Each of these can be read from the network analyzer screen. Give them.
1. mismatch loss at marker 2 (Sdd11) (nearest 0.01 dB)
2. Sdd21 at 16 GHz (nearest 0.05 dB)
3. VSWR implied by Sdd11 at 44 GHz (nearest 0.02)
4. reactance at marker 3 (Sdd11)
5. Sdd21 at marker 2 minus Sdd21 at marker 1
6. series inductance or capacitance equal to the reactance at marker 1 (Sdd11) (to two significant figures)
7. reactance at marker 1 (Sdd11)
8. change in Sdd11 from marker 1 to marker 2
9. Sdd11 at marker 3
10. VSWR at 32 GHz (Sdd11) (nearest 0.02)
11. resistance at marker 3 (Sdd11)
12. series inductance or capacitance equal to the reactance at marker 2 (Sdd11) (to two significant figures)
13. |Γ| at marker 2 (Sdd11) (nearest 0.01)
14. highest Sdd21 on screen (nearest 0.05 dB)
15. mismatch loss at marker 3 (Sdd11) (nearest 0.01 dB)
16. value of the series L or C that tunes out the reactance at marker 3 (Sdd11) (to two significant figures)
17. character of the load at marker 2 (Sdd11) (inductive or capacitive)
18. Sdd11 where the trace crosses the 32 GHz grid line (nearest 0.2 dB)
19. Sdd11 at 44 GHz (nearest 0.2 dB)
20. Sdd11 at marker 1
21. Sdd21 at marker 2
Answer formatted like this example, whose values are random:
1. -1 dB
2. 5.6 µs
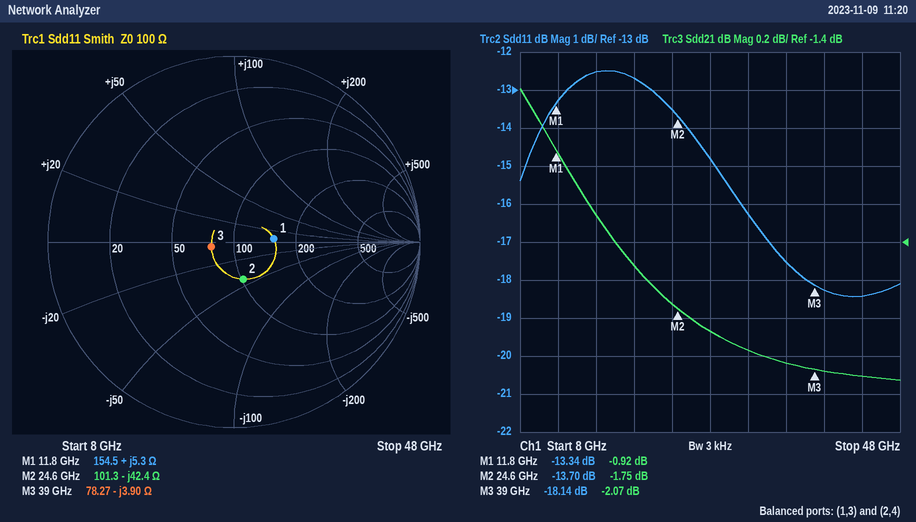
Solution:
1. 0.19 dB
2. -1.25 dB
3. 1.28
4. -3.90 Ω
5. -0.83 dB
6. 71 pH
7. +5.3 Ω
8. -0.36 dB
9. -18.14 dB
10. 1.36
11. 78.27 Ω
12. 150 fF
13. 0.21
14. -0.60 dB
15. 0.07 dB
16. 16 pH
17. capacitive
18. -16.2 dB
19. -18.4 dB
20. -13.34 dB
21. -1.75 dB
